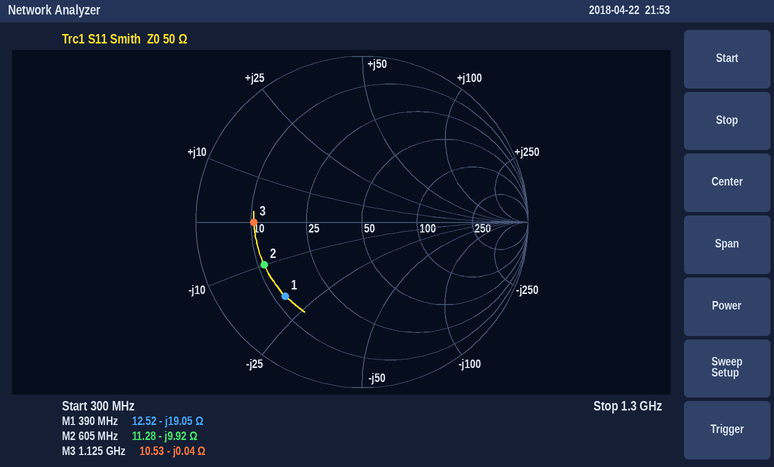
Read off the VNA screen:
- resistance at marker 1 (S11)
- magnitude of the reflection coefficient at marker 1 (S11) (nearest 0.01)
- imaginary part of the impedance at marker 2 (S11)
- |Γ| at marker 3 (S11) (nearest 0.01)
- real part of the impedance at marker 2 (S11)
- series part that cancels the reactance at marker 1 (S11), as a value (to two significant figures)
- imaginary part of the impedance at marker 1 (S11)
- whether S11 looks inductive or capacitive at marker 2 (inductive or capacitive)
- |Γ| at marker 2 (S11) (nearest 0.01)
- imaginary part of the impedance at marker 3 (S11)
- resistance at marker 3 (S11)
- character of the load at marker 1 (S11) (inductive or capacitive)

12.52 Ω
0.64
-9.92 Ω
0.65
11.28 Ω
7.8 nH
-19.05 Ω
capacitive
0.64
-0.04 Ω
10.53 Ω
capacitive
